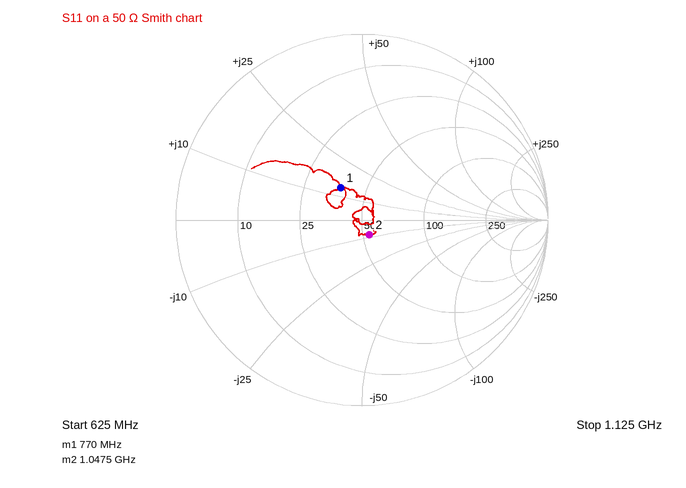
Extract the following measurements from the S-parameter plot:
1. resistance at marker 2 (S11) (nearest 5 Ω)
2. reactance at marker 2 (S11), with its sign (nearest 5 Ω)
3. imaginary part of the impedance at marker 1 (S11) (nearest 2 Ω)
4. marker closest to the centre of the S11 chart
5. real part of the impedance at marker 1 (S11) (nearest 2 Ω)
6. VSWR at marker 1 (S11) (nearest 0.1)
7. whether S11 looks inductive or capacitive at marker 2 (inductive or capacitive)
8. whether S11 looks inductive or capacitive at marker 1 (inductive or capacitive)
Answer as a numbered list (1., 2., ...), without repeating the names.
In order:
1. 55 Ω
2. -10 Ω
3. +14 Ω
4. marker 2
5. 38 Ω
6. 1.5
7. capacitive
8. inductive
